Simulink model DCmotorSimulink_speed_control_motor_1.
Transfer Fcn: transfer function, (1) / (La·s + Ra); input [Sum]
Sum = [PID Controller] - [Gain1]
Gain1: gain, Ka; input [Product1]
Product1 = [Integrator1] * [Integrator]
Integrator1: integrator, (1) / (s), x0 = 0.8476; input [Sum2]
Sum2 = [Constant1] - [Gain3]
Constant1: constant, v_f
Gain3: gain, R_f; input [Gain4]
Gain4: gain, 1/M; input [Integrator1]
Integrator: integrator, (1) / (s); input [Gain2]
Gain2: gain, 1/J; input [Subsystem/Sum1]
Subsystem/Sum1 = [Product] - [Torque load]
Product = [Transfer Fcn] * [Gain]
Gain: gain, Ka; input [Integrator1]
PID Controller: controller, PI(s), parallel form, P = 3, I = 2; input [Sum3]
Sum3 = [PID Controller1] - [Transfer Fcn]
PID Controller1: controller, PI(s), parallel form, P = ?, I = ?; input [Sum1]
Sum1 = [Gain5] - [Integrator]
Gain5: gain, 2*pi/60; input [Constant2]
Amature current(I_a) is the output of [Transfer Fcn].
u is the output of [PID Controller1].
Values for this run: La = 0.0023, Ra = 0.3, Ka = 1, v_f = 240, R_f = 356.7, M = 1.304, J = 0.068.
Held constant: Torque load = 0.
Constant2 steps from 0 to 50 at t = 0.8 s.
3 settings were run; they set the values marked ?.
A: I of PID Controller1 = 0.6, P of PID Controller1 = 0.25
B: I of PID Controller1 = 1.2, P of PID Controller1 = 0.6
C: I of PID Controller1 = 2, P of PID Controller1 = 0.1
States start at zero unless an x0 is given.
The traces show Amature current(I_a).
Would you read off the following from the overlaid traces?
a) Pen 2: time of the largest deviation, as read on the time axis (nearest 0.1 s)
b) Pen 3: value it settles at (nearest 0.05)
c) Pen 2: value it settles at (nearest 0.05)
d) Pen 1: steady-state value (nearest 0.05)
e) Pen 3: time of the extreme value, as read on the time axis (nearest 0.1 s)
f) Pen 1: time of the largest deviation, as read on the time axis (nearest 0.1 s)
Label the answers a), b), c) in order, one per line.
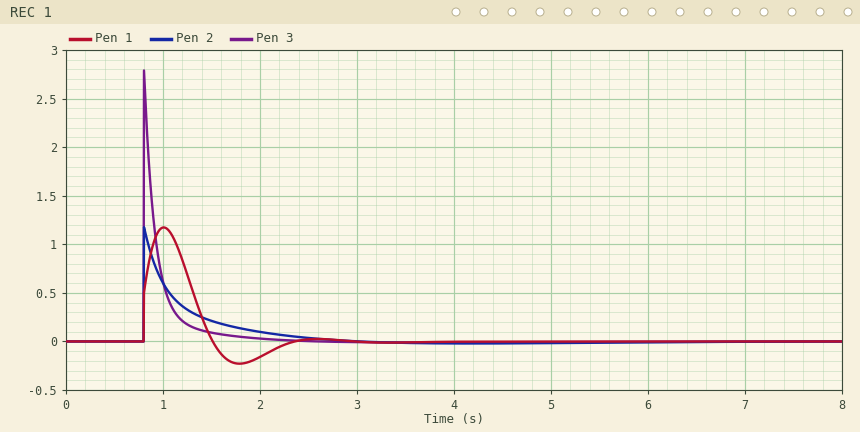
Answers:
a) 0.8 s
b) 0.00
c) 0.00
d) 0.00
e) 0.8 s
f) 1.0 s
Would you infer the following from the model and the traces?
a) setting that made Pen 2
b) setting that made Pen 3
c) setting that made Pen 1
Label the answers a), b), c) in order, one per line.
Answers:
a) A
b) B
c) C
